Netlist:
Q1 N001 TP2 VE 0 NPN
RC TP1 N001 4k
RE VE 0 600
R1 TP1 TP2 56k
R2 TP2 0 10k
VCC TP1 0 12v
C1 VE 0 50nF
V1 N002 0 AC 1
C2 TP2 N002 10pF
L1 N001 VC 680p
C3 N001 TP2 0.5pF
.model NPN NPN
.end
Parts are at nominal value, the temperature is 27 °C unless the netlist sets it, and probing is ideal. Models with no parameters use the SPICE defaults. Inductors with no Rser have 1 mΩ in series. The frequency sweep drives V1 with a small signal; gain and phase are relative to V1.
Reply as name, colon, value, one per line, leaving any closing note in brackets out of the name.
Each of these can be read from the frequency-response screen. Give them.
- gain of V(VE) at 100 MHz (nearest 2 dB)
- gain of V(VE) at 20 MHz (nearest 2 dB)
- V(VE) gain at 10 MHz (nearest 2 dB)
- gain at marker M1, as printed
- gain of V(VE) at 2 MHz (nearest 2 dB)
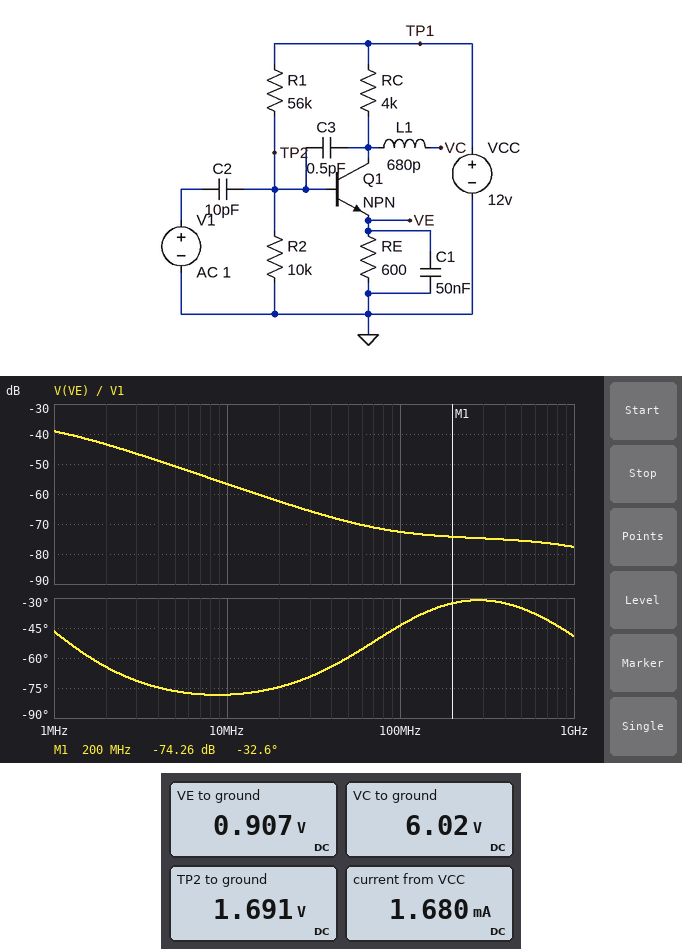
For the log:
gain of V(VE) at 100 MHz: -72 dB
gain of V(VE) at 20 MHz: -62 dB
V(VE) gain at 10 MHz: -56 dB
gain at marker M1, as printed: -74.26 dB
gain of V(VE) at 2 MHz: -44 dB
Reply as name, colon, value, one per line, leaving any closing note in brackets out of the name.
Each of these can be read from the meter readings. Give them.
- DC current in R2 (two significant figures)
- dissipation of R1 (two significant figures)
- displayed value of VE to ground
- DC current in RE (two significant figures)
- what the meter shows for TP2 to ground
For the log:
DC current in R2: 170 µA
dissipation of R1: 1.9 mW
displayed value of VE to ground: 0.907 V
DC current in RE: 1.5 mA
what the meter shows for TP2 to ground: 1.691 V
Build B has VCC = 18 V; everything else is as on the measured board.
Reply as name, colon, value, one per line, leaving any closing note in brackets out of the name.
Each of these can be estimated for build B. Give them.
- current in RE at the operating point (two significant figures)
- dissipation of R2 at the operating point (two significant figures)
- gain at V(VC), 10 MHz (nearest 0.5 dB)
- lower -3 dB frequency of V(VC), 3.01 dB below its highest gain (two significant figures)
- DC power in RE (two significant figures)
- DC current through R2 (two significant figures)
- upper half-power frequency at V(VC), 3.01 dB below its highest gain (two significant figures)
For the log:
current in RE at the operating point: 2.8 mA
dissipation of R2 at the operating point: 620 µW
gain at V(VC), 10 MHz: 25.5 dB
lower -3 dB frequency of V(VC), 3.01 dB below its highest gain: 820 kHz
DC power in RE: 4.8 mW
DC current through R2: 250 µA
upper half-power frequency at V(VC), 3.01 dB below its highest gain: 1.8 GHz
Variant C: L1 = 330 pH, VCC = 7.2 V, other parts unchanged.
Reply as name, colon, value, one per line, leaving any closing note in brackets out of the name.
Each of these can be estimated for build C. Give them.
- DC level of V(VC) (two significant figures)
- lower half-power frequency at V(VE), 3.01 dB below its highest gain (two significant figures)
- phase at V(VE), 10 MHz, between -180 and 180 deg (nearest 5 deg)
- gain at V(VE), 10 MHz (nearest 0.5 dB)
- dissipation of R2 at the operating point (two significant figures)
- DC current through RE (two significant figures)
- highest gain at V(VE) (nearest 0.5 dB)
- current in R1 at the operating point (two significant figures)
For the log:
DC level of V(VC): 5.3 V
lower half-power frequency at V(VE), 3.01 dB below its highest gain: 27 kHz
phase at V(VE), 10 MHz, between -180 and 180 deg: -80 deg
gain at V(VE), 10 MHz: -58.0 dB
dissipation of R2 at the operating point: 110 µW
DC current through RE: 490 µA
highest gain at V(VE): -38.5 dB
current in R1 at the operating point: 110 µA
